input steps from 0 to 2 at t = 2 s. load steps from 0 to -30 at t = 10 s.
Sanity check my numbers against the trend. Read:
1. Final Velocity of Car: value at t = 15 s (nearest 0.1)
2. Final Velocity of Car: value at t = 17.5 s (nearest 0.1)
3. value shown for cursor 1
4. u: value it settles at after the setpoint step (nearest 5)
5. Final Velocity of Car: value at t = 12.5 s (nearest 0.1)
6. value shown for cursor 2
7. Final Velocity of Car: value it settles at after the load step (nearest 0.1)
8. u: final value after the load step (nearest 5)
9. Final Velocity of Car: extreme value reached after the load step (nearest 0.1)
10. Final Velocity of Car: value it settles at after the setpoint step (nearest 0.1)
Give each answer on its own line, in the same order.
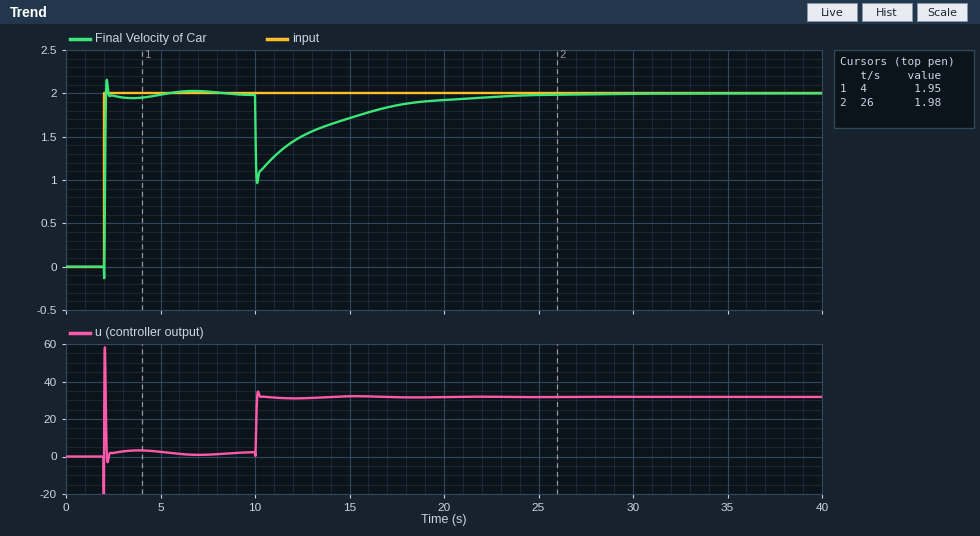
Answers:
1.7
1.9
1.95
0
1.5
1.98
2.0
30
1.0
2.0
